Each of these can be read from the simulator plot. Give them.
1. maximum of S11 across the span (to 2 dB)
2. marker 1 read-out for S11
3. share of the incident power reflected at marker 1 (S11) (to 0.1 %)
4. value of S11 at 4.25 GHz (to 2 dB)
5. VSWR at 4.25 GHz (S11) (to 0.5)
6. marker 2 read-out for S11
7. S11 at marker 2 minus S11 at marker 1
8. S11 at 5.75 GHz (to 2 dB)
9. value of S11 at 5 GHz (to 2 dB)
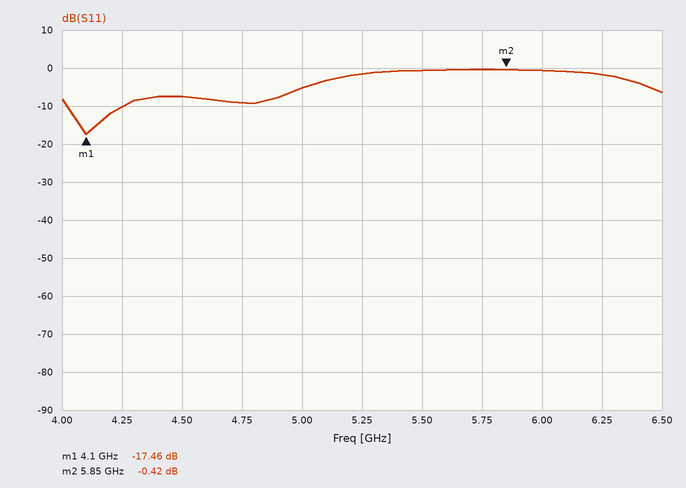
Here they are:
0 dB
-17.46 dB
1.8 %
-10 dB
2.0
-0.42 dB
17.04 dB
0 dB
-6 dB
